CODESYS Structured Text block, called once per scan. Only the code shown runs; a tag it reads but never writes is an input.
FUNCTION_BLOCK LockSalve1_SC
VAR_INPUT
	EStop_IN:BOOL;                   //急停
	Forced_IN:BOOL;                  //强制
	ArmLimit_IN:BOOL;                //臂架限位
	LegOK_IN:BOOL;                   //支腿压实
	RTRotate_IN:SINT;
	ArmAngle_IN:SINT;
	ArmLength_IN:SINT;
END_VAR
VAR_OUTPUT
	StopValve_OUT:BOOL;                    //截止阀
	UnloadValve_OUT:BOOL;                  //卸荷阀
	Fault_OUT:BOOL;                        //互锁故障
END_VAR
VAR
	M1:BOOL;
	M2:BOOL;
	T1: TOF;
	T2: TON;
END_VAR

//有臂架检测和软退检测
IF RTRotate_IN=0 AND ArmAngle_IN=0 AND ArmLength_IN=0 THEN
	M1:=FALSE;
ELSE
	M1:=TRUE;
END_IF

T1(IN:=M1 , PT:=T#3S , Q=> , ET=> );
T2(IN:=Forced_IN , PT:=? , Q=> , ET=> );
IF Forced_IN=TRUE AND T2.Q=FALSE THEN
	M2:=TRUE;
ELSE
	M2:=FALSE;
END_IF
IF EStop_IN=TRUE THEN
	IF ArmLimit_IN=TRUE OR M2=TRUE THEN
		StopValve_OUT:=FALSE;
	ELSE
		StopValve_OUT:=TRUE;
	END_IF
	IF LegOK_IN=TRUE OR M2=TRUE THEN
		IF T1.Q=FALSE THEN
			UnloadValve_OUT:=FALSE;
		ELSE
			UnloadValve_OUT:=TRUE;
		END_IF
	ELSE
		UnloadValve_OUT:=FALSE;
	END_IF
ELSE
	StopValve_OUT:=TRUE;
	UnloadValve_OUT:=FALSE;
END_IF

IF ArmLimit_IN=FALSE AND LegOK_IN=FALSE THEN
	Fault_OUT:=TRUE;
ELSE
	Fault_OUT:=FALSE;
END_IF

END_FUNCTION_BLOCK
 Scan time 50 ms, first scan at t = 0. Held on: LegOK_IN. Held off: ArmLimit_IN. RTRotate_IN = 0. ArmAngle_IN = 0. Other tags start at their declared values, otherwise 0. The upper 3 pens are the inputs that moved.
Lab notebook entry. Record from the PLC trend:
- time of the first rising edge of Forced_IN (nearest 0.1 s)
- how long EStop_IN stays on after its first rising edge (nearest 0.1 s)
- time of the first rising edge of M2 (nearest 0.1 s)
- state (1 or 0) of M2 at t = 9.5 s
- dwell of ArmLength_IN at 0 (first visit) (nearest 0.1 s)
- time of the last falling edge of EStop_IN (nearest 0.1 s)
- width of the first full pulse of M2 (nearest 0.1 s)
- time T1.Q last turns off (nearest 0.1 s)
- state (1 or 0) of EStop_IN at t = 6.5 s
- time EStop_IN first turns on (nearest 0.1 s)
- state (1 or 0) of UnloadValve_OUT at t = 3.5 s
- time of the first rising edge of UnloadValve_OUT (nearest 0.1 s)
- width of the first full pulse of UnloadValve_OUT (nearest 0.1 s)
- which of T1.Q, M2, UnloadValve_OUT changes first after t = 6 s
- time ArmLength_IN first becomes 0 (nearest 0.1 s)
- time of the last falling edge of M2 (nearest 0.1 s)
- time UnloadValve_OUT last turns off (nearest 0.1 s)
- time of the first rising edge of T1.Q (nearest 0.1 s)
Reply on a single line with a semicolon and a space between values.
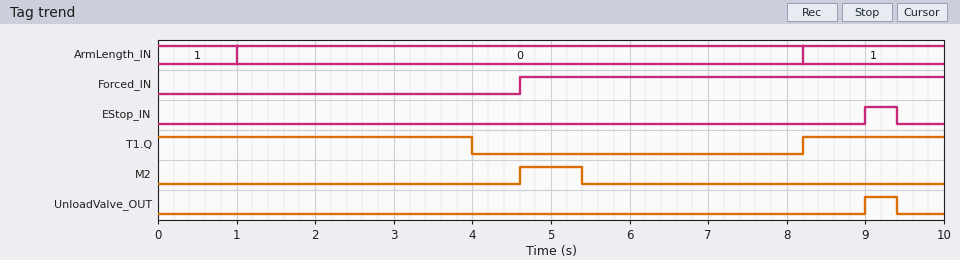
4.6 s; 0.4 s; 4.6 s; 0; 7.2 s; 9.4 s; 0.8 s; 4.0 s; 0; 9.0 s; 0; 9.0 s; 0.4 s; T1.Q; 1.0 s; 5.4 s; 9.4 s; 8.2 s
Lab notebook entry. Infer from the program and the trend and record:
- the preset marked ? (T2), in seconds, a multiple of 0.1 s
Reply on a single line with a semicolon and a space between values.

0.8 s
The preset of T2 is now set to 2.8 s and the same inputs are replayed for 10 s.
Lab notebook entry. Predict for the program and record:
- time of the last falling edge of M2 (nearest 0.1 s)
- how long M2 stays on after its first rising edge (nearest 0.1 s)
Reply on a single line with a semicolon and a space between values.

7.4 s; 2.8 s
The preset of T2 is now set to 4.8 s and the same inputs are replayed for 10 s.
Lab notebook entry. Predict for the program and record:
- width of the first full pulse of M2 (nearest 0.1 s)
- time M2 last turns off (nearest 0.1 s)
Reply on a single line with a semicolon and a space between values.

4.8 s; 9.4 s
